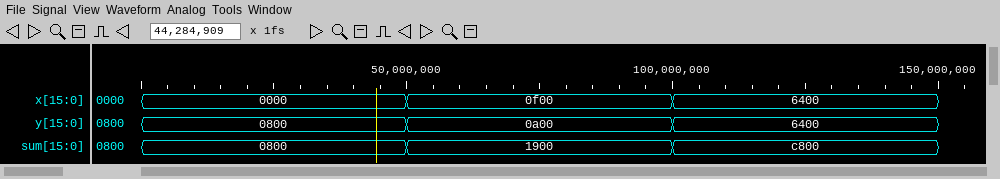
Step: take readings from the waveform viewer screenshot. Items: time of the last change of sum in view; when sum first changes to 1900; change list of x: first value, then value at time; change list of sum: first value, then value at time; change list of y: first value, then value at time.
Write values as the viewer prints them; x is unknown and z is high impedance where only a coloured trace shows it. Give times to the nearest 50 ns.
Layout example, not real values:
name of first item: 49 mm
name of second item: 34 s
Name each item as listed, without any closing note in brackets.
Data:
time of the last change of sum in view: 100 ns
when sum first changes to 1900: 50 ns
change list of x: first value, then value at time: 0000, 0f00 at 50 ns, 6400 at 100 ns
change list of sum: first value, then value at time: 0800, 1900 at 50 ns, c800 at 100 ns
change list of y: first value, then value at time: 0800, 0a00 at 50 ns, 6400 at 100 ns
